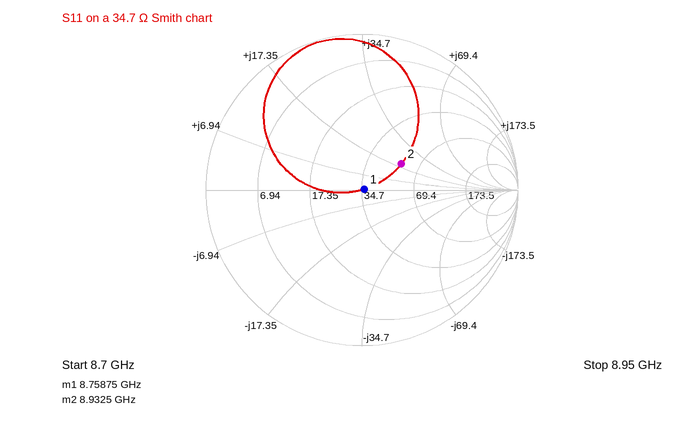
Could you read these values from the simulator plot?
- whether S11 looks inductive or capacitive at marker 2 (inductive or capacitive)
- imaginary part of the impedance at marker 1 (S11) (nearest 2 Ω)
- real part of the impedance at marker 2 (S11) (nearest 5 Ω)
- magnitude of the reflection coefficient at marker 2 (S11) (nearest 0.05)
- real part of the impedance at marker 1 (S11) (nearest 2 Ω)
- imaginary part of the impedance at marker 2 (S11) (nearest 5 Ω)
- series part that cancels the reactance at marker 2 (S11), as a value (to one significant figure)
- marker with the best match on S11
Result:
inductive
0 Ω
55 Ω
0.30
36 Ω
+20 Ω
900 fF
marker 1
